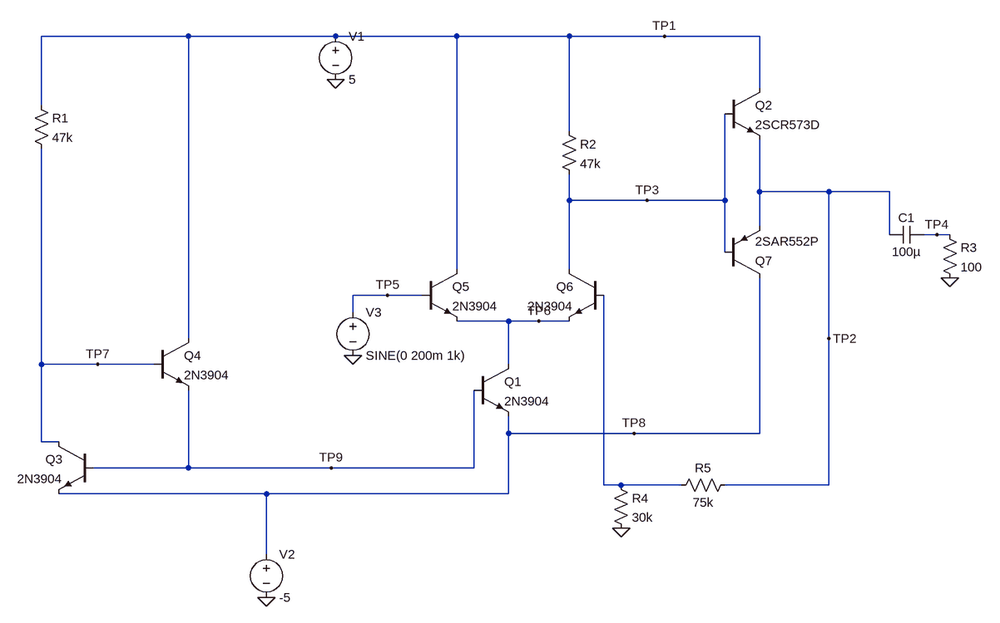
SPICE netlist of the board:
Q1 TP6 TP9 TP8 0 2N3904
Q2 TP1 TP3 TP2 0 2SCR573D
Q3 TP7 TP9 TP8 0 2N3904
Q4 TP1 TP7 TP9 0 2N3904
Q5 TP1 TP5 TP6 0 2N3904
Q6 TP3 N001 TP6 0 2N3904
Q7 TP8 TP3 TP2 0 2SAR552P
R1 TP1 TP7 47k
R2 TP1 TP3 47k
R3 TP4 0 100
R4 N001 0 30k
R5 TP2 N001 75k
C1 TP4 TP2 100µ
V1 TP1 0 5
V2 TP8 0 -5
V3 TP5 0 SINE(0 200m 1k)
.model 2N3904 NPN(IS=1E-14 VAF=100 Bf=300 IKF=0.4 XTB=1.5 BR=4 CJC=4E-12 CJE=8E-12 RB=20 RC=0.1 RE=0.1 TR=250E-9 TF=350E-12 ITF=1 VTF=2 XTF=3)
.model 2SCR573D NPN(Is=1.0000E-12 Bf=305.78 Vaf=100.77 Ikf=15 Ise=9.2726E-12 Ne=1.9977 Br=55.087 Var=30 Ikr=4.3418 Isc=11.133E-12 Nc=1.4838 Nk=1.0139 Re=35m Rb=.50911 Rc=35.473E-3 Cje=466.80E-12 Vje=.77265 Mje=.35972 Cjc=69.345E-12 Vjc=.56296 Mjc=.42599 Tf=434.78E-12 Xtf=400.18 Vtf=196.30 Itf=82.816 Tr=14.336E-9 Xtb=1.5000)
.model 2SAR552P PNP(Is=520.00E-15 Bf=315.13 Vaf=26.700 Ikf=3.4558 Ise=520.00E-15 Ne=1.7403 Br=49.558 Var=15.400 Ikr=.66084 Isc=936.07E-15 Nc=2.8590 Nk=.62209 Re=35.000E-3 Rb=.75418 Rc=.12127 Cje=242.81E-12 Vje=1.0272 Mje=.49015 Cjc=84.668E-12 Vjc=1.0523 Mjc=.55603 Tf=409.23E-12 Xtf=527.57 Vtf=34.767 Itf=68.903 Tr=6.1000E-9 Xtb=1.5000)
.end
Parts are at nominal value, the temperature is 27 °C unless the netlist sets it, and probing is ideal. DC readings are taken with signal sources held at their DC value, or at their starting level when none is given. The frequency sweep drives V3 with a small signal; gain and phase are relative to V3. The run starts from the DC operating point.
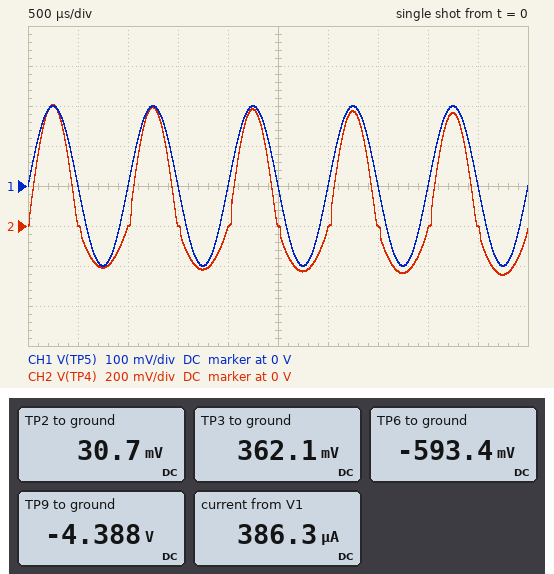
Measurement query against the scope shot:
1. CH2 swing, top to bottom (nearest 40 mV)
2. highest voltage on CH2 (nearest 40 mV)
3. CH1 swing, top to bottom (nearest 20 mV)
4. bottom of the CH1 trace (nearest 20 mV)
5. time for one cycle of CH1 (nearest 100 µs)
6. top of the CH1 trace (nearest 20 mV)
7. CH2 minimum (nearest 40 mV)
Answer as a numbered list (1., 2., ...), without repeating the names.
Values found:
1. 840 mV
2. 600 mV
3. 400 mV
4. -200 mV
5. 1.0 ms
6. 200 mV
7. -240 mV
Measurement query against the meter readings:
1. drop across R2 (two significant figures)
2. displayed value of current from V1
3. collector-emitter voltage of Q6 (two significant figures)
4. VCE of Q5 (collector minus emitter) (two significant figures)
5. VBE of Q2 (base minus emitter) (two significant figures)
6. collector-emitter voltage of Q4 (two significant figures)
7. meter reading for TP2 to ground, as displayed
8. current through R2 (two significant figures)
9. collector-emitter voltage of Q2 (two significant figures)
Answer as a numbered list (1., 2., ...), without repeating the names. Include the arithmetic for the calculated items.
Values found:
1. 5 V - 362.1 mV = 4.6 V
2. 386.3 µA
3. 362.1 mV - (-593.4 mV) = 960 mV
4. 5 V - (-593.4 mV) = 5.6 V
5. 362.1 mV - 30.7 mV = 330 mV
6. 5 V - (-4.388 V) = 9.4 V
7. 30.7 mV
8. (5 V - 362.1 mV) / 47 kΩ = 99 µA
9. 5 V - 30.7 mV = 5.0 V
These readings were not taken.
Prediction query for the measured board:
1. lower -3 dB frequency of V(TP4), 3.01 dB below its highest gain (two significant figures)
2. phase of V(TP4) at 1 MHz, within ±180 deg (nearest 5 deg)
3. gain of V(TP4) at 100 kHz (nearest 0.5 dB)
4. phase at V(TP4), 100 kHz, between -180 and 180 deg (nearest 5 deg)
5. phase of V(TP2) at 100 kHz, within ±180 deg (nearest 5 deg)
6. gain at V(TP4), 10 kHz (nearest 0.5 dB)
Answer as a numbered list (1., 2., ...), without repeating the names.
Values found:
1. 820 mHz
2. -25 deg
3. -18.0 dB
4. -5 deg
5. -5 deg
6. -18.0 dB
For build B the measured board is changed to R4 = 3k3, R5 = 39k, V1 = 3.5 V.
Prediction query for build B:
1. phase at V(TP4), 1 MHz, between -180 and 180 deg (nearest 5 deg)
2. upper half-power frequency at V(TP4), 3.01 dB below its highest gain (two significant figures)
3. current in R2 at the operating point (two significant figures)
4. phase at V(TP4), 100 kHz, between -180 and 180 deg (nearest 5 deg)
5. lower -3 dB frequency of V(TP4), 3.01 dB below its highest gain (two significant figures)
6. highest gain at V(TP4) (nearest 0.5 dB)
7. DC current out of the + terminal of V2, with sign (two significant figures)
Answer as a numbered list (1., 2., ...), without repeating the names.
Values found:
1. -10 deg
2. 4.8 MHz
3. 78 µA
4. 0 deg
5. 4.3 kHz
6. -17.5 dB
7. -320 µA
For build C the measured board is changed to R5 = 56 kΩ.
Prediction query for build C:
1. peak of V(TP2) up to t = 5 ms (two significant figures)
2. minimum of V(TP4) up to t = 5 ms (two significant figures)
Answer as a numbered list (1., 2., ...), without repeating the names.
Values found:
1. 540 mV
2. -230 mV
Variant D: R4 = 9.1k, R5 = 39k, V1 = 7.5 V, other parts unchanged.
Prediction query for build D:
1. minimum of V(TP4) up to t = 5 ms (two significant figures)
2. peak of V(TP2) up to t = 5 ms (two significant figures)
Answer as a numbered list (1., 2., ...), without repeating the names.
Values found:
1. -330 mV
2. 1.0 V
